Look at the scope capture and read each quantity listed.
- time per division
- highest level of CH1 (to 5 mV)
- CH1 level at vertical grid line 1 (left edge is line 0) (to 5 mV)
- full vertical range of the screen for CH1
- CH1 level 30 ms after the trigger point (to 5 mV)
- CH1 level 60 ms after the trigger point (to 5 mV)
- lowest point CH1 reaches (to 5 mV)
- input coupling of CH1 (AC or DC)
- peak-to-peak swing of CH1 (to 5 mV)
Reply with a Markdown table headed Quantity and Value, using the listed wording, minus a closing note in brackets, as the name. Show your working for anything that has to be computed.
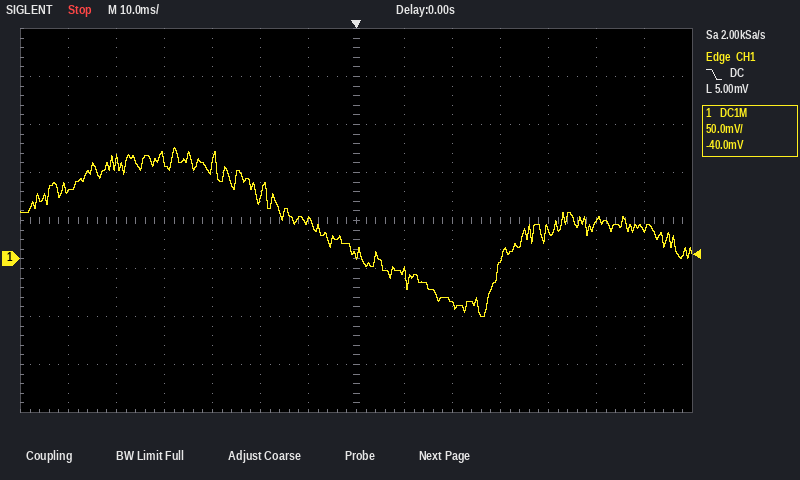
| Quantity | Value |
|---|---|
| time per division | 10 ms |
| highest level of CH1 | 115 mV |
| CH1 level at vertical grid line 1 (left edge is line 0) | 70 mV |
| full vertical range of the screen for CH1 | 400 mV |
| CH1 level 30 ms after the trigger point | 0 mV |
| CH1 level 60 ms after the trigger point | 30 mV |
| lowest point CH1 reaches | -60 mV |
| input coupling of CH1 | DC |
| peak-to-peak swing of CH1 | 115 mV − (-60 mV) = 175 mV |
